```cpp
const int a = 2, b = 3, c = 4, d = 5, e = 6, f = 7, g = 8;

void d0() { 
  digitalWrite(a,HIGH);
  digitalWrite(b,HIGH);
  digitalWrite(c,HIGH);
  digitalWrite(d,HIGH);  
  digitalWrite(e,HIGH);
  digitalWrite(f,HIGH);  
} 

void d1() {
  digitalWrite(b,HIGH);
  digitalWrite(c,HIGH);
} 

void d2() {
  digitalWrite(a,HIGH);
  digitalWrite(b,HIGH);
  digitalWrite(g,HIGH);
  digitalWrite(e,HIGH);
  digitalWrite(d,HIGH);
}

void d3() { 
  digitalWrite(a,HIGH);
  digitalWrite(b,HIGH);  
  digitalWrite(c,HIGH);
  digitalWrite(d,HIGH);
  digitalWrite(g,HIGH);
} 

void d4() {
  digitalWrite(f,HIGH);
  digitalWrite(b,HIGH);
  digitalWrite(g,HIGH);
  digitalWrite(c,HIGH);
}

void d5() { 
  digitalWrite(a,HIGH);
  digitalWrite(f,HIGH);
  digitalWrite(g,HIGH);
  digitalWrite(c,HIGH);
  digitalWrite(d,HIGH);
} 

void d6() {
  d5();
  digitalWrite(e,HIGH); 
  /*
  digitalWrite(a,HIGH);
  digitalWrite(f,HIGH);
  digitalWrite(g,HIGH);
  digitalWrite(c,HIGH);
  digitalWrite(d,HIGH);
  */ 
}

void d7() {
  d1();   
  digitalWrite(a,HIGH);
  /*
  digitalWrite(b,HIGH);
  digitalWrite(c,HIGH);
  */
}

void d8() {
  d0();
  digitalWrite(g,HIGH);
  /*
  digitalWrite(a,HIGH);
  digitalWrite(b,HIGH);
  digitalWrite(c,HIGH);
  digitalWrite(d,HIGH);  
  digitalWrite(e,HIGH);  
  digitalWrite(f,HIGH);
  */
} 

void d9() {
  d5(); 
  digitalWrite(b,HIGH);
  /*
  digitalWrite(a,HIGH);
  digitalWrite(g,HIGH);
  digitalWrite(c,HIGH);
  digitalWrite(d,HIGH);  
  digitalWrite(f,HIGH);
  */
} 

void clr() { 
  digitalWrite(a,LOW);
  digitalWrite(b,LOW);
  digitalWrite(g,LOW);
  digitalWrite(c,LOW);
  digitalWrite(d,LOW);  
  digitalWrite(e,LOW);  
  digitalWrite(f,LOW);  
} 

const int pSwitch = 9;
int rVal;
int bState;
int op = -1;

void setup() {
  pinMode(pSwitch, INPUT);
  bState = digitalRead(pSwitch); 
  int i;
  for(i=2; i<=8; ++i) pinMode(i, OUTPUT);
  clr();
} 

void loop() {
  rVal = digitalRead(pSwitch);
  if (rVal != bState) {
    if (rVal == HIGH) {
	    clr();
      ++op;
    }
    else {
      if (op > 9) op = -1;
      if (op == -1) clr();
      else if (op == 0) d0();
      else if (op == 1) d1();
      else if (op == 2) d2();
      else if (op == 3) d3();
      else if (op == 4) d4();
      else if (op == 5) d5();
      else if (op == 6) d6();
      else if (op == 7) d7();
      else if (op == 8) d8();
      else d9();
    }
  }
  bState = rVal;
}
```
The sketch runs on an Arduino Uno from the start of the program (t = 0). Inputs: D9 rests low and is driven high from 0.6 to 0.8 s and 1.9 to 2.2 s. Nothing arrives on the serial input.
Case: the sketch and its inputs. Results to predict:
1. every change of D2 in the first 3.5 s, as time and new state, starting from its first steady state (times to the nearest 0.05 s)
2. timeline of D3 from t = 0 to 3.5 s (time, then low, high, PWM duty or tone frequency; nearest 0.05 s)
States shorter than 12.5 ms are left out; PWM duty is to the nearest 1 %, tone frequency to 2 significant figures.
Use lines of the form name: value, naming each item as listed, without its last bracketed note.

every change of D2 in the first 3.5 s, as time and new state, starting from its first steady state: 0 s low; 0.8 s high; 1.9 s low
timeline of D3 from t = 0 to 3.5 s: 0 s low; 0.8 s high; 1.9 s low; 2.2 s high
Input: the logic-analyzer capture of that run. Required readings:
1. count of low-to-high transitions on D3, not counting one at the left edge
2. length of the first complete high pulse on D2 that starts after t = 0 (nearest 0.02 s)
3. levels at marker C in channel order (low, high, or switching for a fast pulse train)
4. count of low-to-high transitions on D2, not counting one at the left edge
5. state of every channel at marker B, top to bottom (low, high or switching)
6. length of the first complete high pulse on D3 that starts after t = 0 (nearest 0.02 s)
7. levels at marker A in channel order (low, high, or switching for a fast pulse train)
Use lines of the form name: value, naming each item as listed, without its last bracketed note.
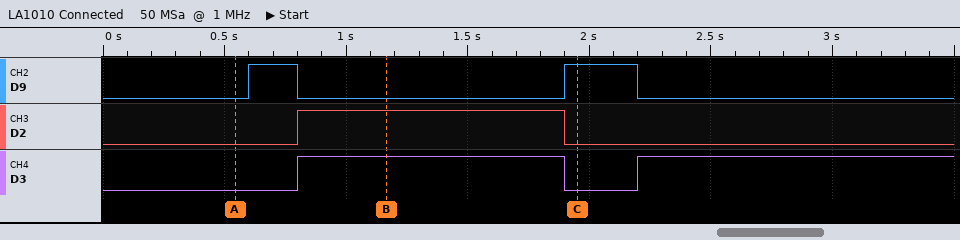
count of low-to-high transitions on D3, not counting one at the left edge: 2
length of the first complete high pulse on D2 that starts after t = 0: 1.10 s
levels at marker C in channel order: D9 high, D2 low, D3 low
count of low-to-high transitions on D2, not counting one at the left edge: 1
state of every channel at marker B, top to bottom: D9 low, D2 high, D3 high
length of the first complete high pulse on D3 that starts after t = 0: 1.10 s
levels at marker A in channel order: D9 low, D2 low, D3 low
